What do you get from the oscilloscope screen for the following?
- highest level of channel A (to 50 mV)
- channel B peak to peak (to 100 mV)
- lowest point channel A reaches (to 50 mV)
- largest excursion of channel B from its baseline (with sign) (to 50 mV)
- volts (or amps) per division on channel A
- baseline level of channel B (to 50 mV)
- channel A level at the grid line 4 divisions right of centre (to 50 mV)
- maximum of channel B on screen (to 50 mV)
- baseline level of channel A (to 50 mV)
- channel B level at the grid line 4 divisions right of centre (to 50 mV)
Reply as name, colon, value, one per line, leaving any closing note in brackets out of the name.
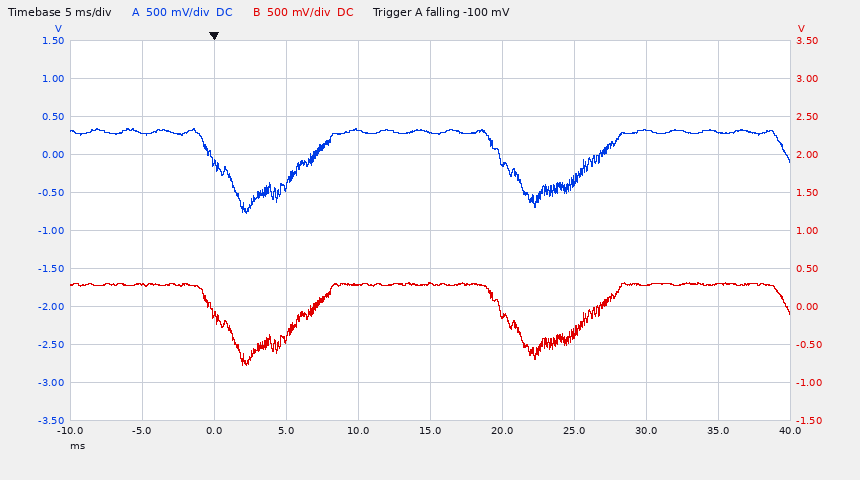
highest level of channel A: 350 mV
channel B peak to peak: 1.10 V
lowest point channel A reaches: -800 mV
largest excursion of channel B from its baseline (with sign): -1.05 V
volts (or amps) per division on channel A: 500 mV
baseline level of channel B: 300 mV
channel A level at the grid line 4 divisions right of centre: 300 mV
maximum of channel B on screen: 300 mV
baseline level of channel A: 300 mV
channel B level at the grid line 4 divisions right of centre: 300 mV
